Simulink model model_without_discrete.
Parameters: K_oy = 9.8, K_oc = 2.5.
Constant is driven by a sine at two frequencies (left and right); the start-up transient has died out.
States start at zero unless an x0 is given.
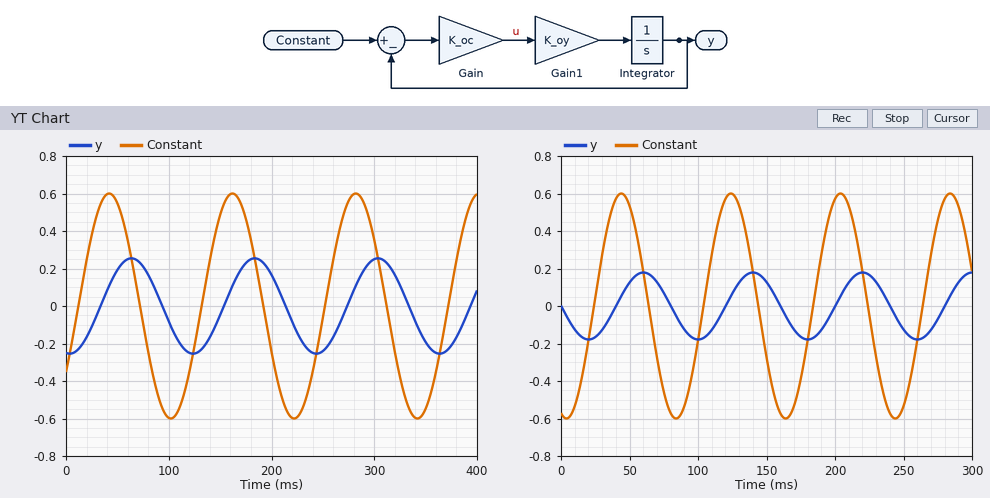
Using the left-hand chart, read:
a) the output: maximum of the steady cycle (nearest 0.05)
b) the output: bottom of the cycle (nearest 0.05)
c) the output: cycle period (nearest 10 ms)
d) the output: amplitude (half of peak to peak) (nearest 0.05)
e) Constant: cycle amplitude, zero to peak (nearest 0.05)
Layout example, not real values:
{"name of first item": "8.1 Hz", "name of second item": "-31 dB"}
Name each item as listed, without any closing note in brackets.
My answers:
{"the output: maximum of the steady cycle": "0.25", "the output: bottom of the cycle": "-0.25", "the output: cycle period": "120 ms", "the output: amplitude (half of peak to peak)": "0.25", "Constant: cycle amplitude, zero to peak": "0.60"}
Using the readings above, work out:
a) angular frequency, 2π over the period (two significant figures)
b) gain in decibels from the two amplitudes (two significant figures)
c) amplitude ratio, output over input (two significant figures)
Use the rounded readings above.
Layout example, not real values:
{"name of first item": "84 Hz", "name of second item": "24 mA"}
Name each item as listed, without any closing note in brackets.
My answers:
{"angular frequency, 2π over the period": "0.052 rad/ms", "gain in decibels from the two amplitudes": "-7.6 dB", "amplitude ratio, output over input": "0.42"}
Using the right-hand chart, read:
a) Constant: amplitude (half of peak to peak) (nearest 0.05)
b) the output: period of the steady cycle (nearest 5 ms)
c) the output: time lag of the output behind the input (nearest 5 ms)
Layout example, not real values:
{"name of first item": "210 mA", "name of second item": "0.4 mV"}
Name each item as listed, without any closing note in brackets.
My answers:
{"Constant: amplitude (half of peak to peak)": "0.60", "the output: period of the steady cycle": "80 ms", "the output: time lag of the output behind the input": "15 ms"}
